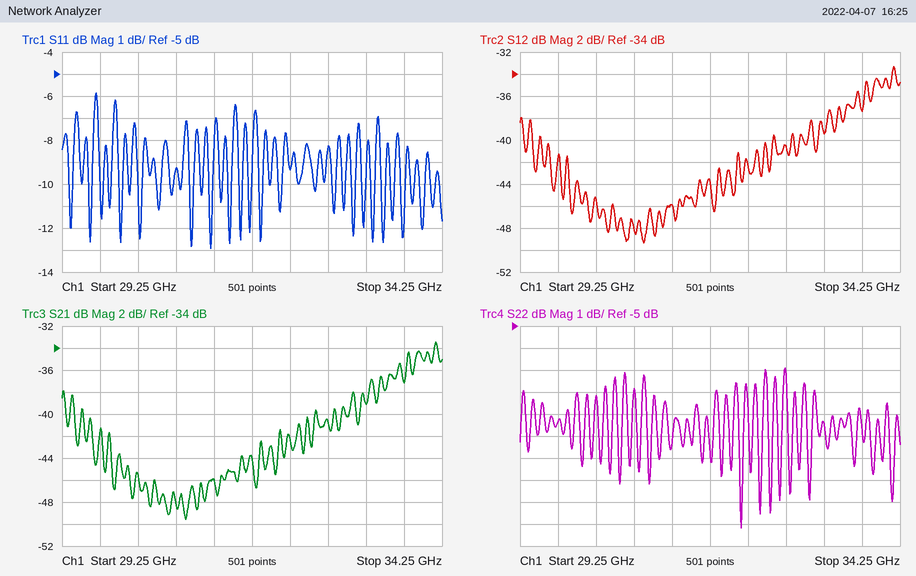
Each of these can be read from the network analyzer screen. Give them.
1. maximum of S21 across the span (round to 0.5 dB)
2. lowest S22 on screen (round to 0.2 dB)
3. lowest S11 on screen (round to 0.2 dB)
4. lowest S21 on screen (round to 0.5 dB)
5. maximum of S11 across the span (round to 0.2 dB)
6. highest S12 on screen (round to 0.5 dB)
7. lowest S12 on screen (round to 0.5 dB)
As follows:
-33.5 dB
-14.2 dB
-13.0 dB
-49.5 dB
-5.8 dB
-33.5 dB
-49.5 dB
